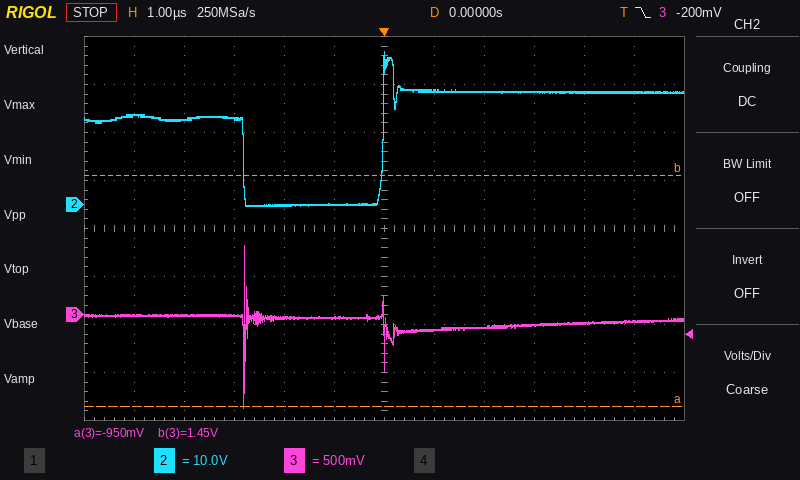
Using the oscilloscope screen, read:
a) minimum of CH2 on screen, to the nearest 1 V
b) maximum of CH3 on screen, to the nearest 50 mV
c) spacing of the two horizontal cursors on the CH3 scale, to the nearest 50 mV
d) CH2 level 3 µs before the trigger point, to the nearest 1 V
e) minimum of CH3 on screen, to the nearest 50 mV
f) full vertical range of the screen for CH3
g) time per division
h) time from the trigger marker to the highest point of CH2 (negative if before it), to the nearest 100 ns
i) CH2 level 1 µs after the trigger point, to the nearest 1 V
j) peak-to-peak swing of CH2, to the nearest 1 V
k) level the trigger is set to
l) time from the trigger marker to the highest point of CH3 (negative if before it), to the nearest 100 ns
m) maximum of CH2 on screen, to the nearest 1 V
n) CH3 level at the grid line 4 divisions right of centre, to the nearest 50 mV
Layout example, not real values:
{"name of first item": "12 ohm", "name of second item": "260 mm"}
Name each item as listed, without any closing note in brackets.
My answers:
{"minimum of CH2 on screen, to the nearest 1 V": "0 V", "maximum of CH3 on screen, to the nearest 50 mV": "700 mV", "spacing of the two horizontal cursors on the CH3 scale, to the nearest 50 mV": "2.40 V", "CH2 level 3 µs before the trigger point, to the nearest 1 V": "18 V", "minimum of CH3 on screen, to the nearest 50 mV": "-950 mV", "full vertical range of the screen for CH3": "4 V", "time per division": "1 µs", "time from the trigger marker to the highest point of CH2 (negative if before it), to the nearest 100 ns": "0.0 µs", "CH2 level 1 µs after the trigger point, to the nearest 1 V": "24 V", "peak-to-peak swing of CH2, to the nearest 1 V": "32 V", "level the trigger is set to": "-200 mV", "time from the trigger marker to the highest point of CH3 (negative if before it), to the nearest 100 ns": "-2.8 µs", "maximum of CH2 on screen, to the nearest 1 V": "32 V", "CH3 level at the grid line 4 divisions right of centre, to the nearest 50 mV": "-100 mV"}
